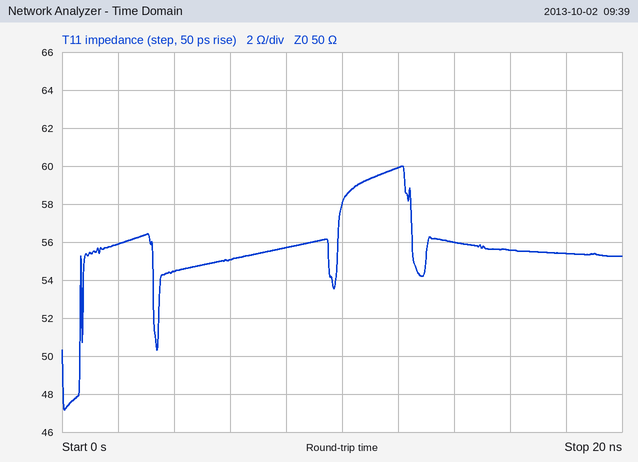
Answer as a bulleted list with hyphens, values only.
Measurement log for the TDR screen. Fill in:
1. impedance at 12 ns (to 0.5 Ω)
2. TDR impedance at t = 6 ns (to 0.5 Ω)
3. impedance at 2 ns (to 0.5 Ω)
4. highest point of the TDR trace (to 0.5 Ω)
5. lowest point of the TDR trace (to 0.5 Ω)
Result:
- 60.0 Ω
- 55.0 Ω
- 56.0 Ω
- 60.0 Ω
- 47.0 Ω
